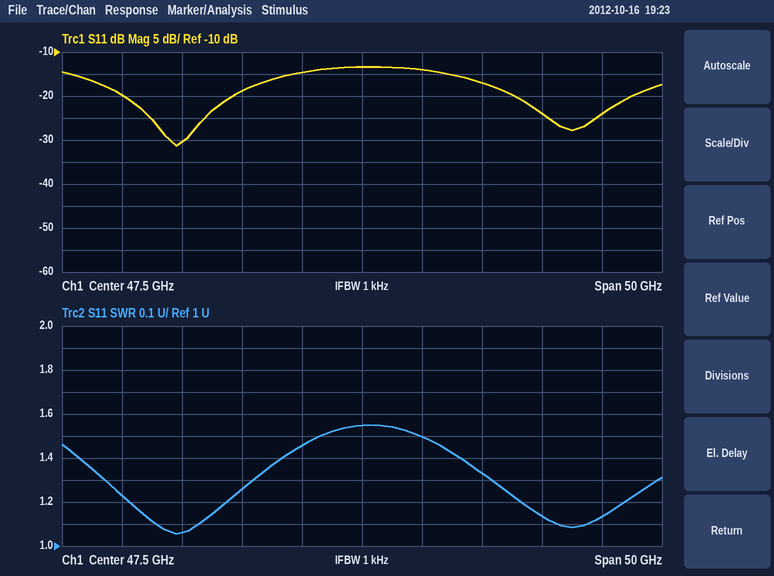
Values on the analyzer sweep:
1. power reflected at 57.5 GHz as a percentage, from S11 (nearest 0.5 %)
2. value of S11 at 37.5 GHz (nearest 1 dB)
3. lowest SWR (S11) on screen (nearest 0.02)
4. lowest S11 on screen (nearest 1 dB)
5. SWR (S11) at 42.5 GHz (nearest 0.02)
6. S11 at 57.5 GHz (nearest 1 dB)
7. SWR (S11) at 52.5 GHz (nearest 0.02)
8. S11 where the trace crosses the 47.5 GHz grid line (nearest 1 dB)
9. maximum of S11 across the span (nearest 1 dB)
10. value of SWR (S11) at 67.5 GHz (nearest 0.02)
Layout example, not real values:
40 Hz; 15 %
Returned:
2.0 %; -19 dB; 1.06; -31 dB; 1.46; -17 dB; 1.50; -13 dB; -13 dB; 1.14
